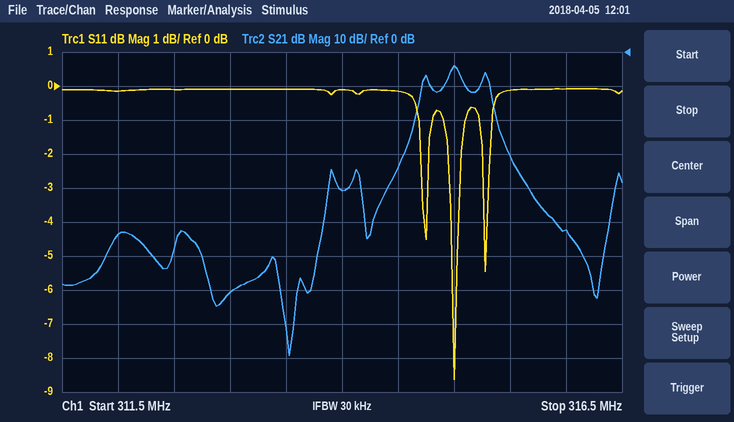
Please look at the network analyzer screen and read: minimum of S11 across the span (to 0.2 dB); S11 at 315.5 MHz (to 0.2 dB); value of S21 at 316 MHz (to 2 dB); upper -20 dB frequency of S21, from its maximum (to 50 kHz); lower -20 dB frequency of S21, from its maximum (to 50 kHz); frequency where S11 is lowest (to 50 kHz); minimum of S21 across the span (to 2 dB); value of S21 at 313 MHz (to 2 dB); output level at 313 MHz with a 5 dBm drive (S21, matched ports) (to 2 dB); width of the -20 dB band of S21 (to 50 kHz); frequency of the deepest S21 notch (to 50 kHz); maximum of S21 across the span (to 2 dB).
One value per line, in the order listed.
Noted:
-8.6 dB
-0.2 dB
-52 dB
315.40 MHz
314.60 MHz
315.00 MHz
-90 dB
-70 dB
-66 dBm
800 kHz
313.55 MHz
-4 dB
